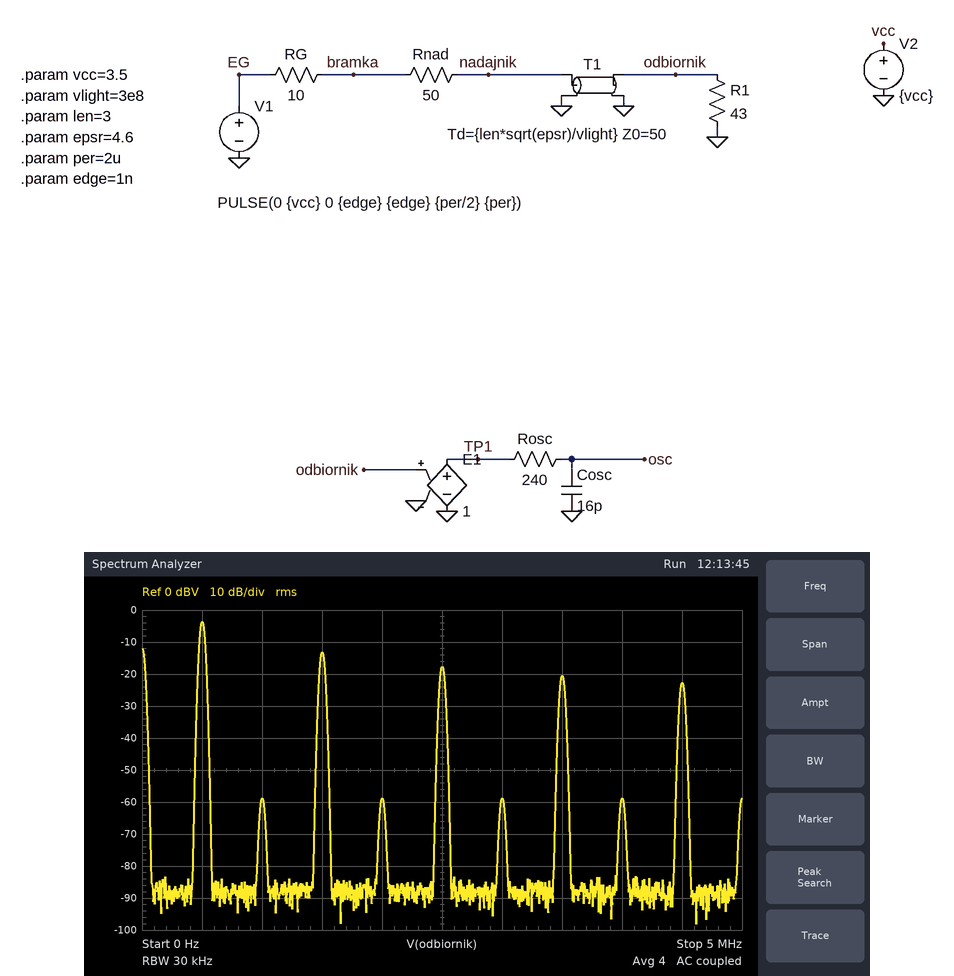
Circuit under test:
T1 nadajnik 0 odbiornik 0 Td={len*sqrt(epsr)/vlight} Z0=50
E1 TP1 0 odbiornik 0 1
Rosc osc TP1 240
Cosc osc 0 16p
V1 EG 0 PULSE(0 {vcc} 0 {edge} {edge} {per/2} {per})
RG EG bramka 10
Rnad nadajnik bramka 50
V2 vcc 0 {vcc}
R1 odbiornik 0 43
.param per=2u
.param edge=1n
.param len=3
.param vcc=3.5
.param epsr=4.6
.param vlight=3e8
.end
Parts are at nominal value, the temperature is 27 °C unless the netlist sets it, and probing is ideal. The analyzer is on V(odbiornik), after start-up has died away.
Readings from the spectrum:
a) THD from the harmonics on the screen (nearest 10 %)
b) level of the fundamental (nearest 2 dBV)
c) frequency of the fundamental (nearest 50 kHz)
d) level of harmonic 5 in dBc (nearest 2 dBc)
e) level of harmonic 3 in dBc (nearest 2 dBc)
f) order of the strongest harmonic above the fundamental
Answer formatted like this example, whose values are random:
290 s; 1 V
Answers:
40 %; -4 dBV; 500 kHz; -14 dBc; -10 dBc; 3
